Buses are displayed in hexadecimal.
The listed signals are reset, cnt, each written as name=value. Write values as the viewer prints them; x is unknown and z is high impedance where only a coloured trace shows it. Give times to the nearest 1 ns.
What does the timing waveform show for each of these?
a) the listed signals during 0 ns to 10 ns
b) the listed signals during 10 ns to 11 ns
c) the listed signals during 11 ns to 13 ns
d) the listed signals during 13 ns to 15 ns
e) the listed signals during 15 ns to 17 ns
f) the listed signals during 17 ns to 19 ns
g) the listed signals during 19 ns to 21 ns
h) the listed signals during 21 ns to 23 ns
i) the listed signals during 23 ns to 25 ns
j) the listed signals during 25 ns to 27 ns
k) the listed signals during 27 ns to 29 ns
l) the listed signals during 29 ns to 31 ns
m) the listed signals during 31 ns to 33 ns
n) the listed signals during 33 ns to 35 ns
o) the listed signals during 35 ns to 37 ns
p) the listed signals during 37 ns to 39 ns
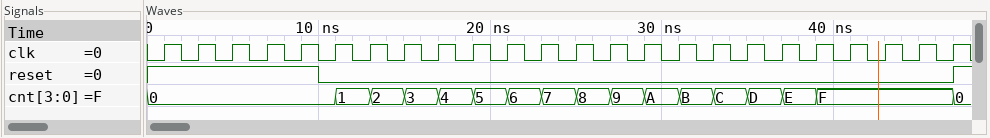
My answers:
reset=1, cnt=0
reset=0, cnt=0
reset=0, cnt=1
reset=0, cnt=2
reset=0, cnt=3
reset=0, cnt=4
reset=0, cnt=5
reset=0, cnt=6
reset=0, cnt=7
reset=0, cnt=8
reset=0, cnt=9
reset=0, cnt=A
reset=0, cnt=B
reset=0, cnt=C
reset=0, cnt=D
reset=0, cnt=E
